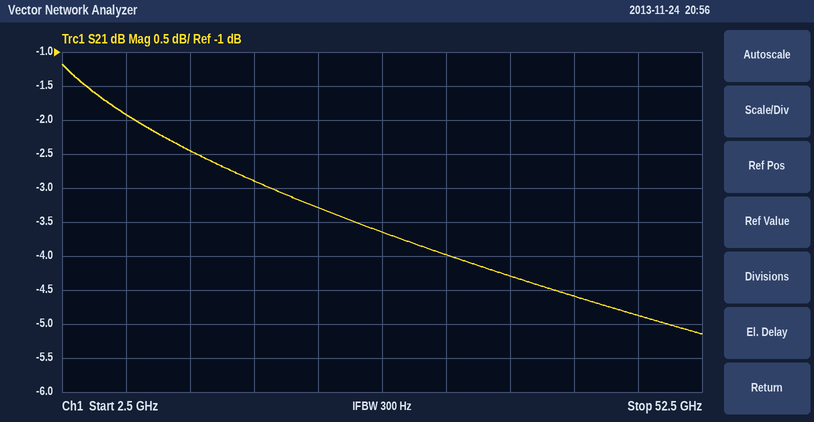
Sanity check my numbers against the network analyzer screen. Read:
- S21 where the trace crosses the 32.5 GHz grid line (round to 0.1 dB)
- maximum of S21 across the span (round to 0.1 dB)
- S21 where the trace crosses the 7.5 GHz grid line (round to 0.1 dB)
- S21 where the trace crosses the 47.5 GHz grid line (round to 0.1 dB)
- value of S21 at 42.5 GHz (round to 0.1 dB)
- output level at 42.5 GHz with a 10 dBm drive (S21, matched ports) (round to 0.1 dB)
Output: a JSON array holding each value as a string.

["-4.0 dB", "-1.2 dB", "-1.9 dB", "-4.9 dB", "-4.6 dB", "5.4 dBm"]
